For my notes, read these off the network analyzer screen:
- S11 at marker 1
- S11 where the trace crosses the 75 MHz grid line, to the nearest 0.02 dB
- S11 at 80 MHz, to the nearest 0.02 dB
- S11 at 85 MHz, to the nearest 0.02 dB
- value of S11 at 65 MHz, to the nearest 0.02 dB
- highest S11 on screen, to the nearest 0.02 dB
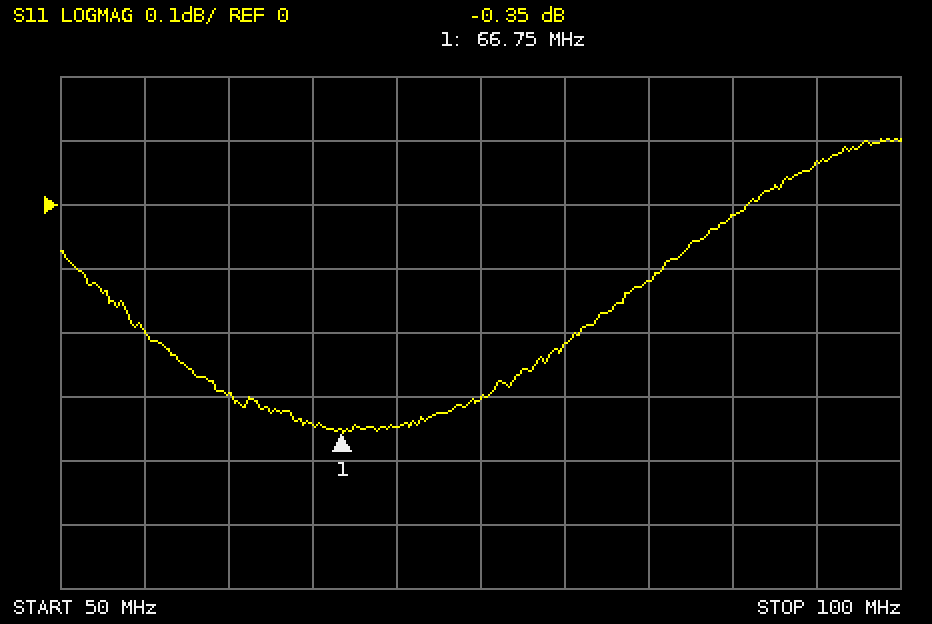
-0.35 dB
-0.30 dB
-0.22 dB
-0.12 dB
-0.34 dB
0.10 dB
